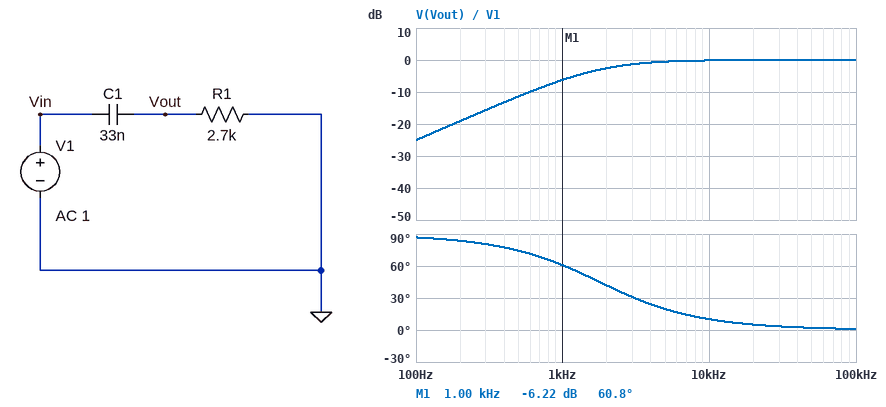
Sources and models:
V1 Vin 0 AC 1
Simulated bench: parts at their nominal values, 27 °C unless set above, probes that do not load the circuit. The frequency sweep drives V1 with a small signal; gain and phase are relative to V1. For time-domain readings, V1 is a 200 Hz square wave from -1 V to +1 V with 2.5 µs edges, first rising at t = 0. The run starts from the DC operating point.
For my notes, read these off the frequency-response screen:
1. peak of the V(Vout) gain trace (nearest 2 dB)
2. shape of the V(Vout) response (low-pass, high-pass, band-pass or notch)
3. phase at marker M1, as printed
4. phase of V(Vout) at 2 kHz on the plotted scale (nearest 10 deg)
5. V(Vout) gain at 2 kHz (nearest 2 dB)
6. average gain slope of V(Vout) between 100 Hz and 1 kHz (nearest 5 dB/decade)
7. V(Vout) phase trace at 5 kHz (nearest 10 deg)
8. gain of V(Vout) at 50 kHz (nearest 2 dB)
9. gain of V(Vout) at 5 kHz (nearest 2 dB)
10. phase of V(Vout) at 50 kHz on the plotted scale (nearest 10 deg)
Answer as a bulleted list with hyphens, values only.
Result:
- 0 dB
- high-pass
- 60.8 deg
- 40 deg
- -2 dB
- 20 dB/decade
- 20 deg
- 0 dB
- 0 dB
- 0 deg
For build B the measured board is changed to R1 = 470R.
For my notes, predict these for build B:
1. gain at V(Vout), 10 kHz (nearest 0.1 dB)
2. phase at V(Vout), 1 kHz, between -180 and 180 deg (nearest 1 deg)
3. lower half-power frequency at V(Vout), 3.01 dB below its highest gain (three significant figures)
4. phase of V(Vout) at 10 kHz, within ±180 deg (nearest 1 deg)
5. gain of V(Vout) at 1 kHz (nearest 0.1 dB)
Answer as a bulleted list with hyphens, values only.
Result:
- -3.1 dB
- 84 deg
- 10.3 kHz
- 46 deg
- -20.3 dB
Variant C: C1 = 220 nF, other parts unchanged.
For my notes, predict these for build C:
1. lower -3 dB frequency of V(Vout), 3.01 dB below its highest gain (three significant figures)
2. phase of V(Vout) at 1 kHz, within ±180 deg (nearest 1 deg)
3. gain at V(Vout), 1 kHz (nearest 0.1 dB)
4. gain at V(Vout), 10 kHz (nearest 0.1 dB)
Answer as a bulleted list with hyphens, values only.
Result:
- 268 Hz
- 15 deg
- -0.3 dB
- 0 dB
